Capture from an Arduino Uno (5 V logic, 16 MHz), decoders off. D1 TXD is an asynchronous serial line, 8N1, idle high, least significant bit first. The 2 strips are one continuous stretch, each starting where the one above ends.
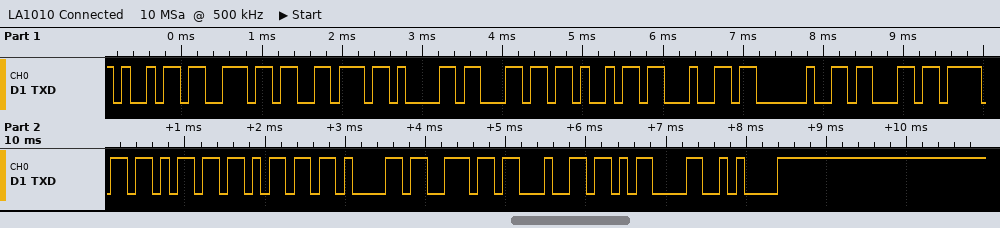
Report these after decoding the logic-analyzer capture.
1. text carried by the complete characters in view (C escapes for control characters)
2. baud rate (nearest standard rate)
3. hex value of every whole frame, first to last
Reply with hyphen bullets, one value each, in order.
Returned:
- "invalid command\r\n"
- 9600 baud
- 69 6E 76 61 6C 69 64 20 63 6F 6D 6D 61 6E 64 0D 0A
